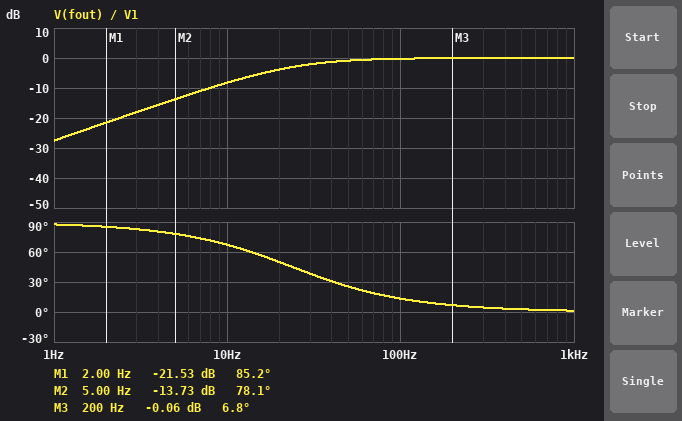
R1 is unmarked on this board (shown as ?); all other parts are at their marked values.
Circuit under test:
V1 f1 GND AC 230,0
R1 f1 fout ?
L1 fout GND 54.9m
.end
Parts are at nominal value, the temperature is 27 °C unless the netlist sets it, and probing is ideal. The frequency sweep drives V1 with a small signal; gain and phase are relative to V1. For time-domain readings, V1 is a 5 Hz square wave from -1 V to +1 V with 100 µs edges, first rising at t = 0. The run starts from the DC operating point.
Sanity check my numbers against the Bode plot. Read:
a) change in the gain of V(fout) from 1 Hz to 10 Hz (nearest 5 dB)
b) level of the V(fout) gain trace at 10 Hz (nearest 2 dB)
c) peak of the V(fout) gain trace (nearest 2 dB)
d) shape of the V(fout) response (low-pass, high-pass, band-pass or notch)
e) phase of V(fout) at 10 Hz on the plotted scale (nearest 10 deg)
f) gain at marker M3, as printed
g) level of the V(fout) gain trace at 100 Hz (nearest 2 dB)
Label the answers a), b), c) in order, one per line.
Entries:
a) 20 dB
b) -8 dB
c) 0 dB
d) high-pass
e) 70 deg
f) -0.06 dB
g) 0 dB
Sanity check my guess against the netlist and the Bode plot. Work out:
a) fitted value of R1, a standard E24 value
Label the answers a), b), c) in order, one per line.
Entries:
a) 8.2 Ω
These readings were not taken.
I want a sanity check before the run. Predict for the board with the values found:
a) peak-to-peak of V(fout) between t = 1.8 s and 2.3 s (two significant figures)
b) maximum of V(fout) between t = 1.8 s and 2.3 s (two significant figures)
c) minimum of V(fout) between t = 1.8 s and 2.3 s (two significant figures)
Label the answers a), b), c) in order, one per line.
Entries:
a) 4.0 V
b) 2.0 V
c) -2.0 V
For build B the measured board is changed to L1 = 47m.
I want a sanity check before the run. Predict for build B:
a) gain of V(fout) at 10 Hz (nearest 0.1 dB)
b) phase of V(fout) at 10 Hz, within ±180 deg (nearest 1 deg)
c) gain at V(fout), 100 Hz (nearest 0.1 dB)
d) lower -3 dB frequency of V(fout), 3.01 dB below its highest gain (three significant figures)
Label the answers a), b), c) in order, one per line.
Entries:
a) -9.4 dB
b) 70 deg
c) -0.3 dB
d) 27.8 Hz
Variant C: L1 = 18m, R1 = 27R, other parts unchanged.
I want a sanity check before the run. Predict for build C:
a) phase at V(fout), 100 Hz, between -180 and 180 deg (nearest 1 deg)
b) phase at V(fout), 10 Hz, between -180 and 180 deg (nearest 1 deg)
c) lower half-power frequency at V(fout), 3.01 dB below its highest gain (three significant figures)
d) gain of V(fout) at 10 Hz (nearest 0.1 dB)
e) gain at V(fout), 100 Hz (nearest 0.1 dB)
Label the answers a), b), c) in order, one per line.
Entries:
a) 67 deg
b) 88 deg
c) 239 Hz
d) -27.6 dB
e) -8.3 dB
